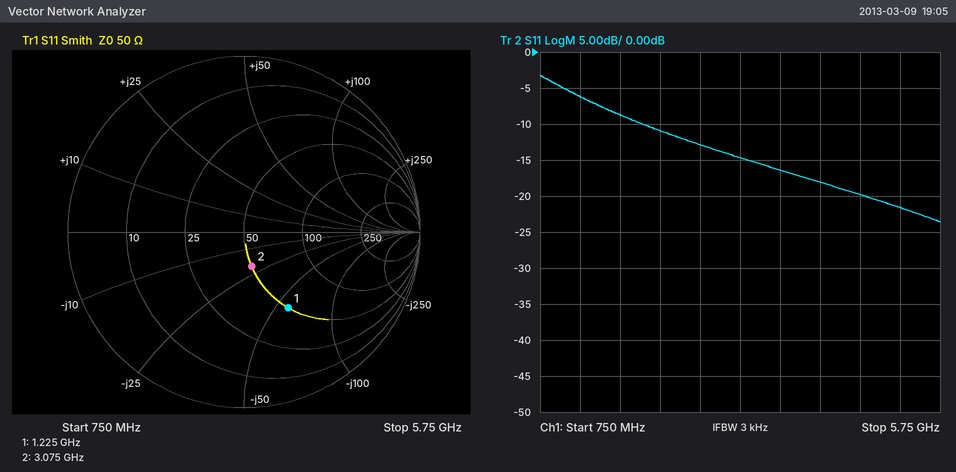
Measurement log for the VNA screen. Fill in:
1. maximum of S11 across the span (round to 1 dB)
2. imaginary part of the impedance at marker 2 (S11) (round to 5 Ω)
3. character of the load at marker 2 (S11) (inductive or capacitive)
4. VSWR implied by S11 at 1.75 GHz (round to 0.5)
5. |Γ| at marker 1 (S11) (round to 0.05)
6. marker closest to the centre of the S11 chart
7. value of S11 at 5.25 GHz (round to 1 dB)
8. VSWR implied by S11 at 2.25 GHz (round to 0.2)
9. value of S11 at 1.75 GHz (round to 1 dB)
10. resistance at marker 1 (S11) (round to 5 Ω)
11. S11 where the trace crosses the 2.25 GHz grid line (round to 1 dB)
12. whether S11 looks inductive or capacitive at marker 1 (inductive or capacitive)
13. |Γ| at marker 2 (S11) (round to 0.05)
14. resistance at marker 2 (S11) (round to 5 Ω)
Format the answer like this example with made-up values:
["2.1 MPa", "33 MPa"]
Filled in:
["-3 dB", "-20 Ω", "capacitive", "2.0", "0.50", "marker 2", "-22 dB", "1.8", "-9 dB", "50 Ω", "-11 dB", "capacitive", "0.20", "50 Ω"]
